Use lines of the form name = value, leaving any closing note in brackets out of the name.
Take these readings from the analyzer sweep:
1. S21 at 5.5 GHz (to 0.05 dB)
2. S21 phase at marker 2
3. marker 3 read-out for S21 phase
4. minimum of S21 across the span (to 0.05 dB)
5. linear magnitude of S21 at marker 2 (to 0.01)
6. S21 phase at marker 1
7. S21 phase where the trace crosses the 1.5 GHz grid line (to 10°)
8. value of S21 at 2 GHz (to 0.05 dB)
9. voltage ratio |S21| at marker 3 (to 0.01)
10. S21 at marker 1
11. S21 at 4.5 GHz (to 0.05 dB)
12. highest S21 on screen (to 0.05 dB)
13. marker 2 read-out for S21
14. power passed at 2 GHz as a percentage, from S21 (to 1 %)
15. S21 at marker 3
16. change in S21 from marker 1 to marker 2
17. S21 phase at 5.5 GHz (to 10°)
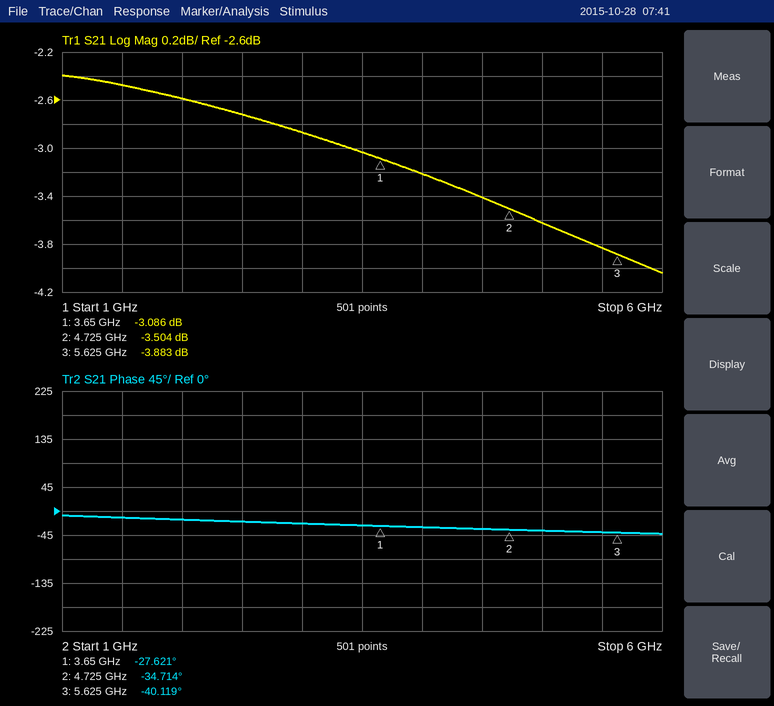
S21 at 5.5 GHz = -3.85 dB
S21 phase at marker 2 = -34.714°
marker 3 read-out for S21 phase = -40.119°
minimum of S21 across the span = -4.05 dB
linear magnitude of S21 at marker 2 = 0.67
S21 phase at marker 1 = -27.621°
S21 phase where the trace crosses the 1.5 GHz grid line = -10°
value of S21 at 2 GHz = -2.60 dB
voltage ratio |S21| at marker 3 = 0.64
S21 at marker 1 = -3.086 dB
S21 at 4.5 GHz = -3.40 dB
highest S21 on screen = -2.40 dB
marker 2 read-out for S21 = -3.504 dB
power passed at 2 GHz as a percentage, from S21 = 55 %
S21 at marker 3 = -3.883 dB
change in S21 from marker 1 to marker 2 = -0.418 dB
S21 phase at 5.5 GHz = -40°
